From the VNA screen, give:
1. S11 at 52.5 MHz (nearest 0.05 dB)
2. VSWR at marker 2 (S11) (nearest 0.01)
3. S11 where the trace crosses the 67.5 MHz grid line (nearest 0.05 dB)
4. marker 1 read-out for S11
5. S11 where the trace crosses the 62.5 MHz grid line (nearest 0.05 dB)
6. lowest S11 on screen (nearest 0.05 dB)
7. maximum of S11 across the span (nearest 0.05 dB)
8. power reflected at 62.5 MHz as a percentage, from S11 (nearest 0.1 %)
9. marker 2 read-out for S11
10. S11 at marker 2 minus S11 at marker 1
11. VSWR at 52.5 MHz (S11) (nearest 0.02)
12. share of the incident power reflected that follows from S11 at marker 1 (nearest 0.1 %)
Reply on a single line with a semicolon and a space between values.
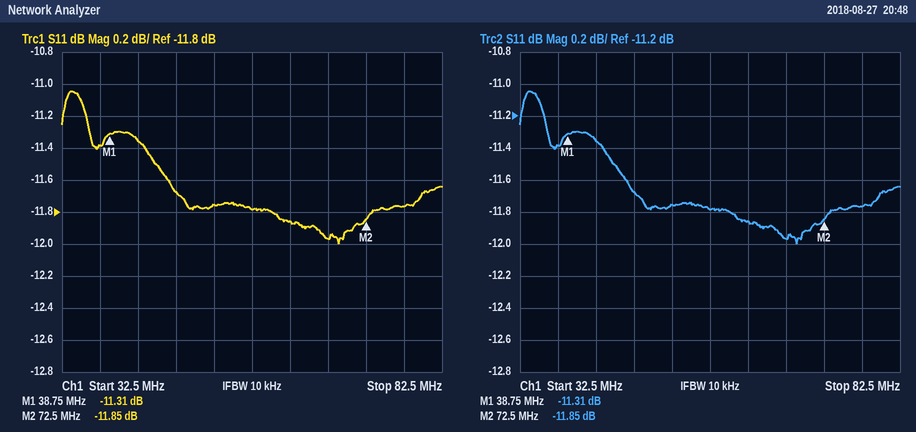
-11.75 dB; 1.69; -11.95 dB; -11.31 dB; -11.85 dB; -12.00 dB; -11.05 dB; 6.5 %; -11.85 dB; -0.54 dB; 1.70; 7.4 %
